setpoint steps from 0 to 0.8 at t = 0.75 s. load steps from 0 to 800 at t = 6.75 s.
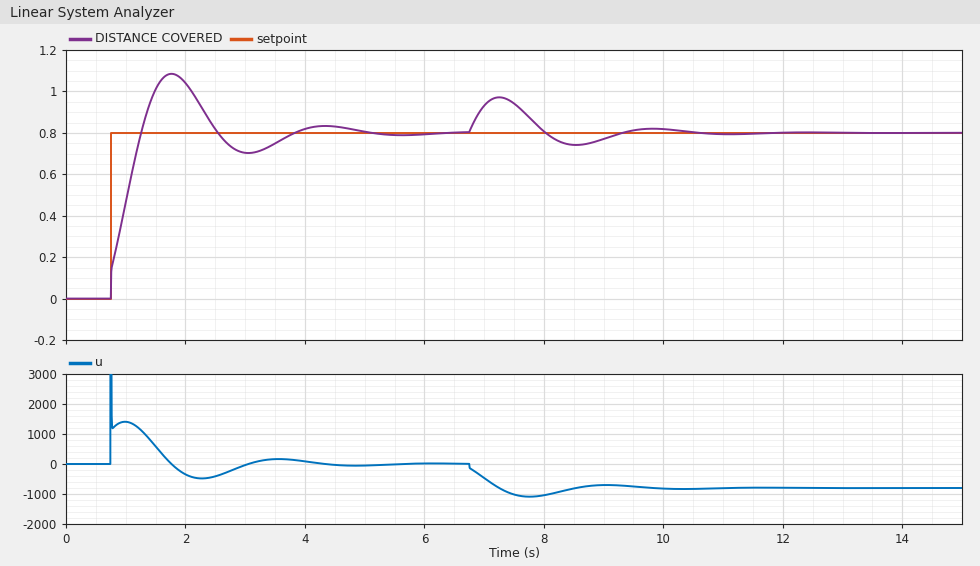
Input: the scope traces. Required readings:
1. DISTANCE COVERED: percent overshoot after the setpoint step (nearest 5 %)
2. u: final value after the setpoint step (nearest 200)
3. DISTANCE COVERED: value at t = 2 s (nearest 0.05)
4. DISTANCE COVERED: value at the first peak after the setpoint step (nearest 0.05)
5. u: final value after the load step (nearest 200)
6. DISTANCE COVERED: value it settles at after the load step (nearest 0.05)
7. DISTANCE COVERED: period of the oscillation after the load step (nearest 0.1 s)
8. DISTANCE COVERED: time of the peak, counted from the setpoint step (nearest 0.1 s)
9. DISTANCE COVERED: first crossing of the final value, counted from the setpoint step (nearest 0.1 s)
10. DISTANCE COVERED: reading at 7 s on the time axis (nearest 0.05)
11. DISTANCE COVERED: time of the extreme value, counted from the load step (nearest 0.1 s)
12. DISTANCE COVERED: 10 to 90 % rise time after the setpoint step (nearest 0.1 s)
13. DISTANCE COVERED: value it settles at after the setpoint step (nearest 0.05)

35 %
0
1.05
1.10
-800
0.80
2.6 s
1.0 s
0.5 s
0.95
0.5 s
0.4 s
0.80
